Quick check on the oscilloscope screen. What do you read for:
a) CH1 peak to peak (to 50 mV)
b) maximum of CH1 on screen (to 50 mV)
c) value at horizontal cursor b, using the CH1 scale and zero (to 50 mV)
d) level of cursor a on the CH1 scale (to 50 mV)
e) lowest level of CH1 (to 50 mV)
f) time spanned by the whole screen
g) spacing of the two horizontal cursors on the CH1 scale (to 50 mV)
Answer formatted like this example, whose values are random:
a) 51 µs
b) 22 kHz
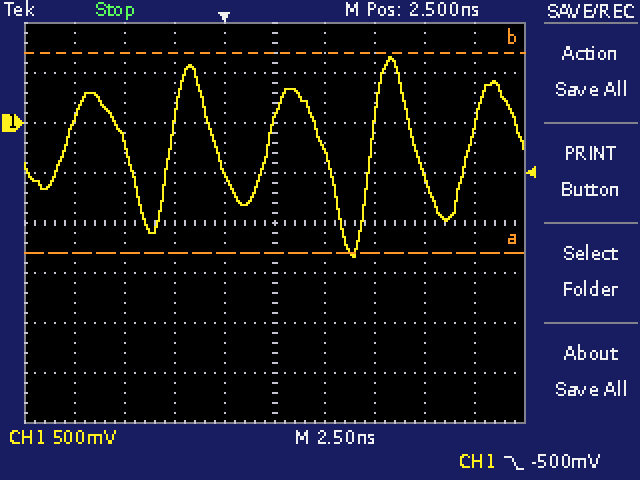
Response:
a) 2.00 V
b) 650 mV
c) 700 mV
d) -1.30 V
e) -1.35 V
f) 25 ns
g) 2.00 V
